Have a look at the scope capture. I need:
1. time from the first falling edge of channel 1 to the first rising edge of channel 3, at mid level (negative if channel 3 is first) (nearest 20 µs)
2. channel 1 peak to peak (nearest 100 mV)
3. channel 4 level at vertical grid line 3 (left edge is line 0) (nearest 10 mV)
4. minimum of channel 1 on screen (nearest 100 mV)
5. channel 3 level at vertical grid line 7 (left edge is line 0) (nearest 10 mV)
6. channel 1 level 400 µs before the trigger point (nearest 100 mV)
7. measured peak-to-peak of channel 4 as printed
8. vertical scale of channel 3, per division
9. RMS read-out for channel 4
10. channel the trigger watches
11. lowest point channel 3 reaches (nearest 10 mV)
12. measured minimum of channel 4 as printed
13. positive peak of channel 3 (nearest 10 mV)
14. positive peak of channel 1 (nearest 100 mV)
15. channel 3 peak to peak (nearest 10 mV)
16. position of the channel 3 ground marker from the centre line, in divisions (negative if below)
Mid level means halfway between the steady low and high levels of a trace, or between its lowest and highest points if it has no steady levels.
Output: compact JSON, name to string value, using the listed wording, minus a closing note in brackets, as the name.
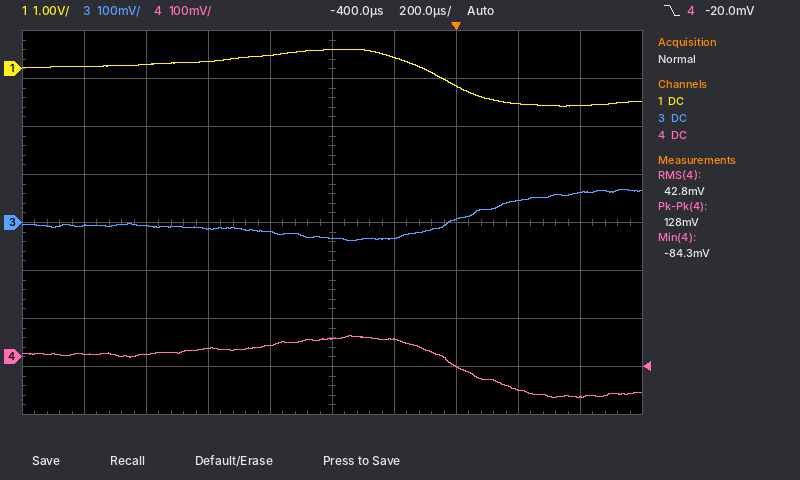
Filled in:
{"time from the first falling edge of channel 1 to the first rising edge of channel 3, at mid level (negative if channel 3 is first)": "+100 µs", "channel 1 peak to peak": "1.2 V", "channel 4 level at vertical grid line 3 (left edge is line 0)": "20 mV", "minimum of channel 1 on screen": "-800 mV", "channel 3 level at vertical grid line 7 (left edge is line 0)": "10 mV", "channel 1 level 400 µs before the trigger point": "400 mV", "measured peak-to-peak of channel 4 as printed": "128 mV", "vertical scale of channel 3, per division": "100 mV", "RMS read-out for channel 4": "42.8 mV", "channel the trigger watches": "channel 4", "lowest point channel 3 reaches": "-40 mV", "measured minimum of channel 4 as printed": "-84.3 mV", "positive peak of channel 3": "70 mV", "positive peak of channel 1": "400 mV", "channel 3 peak to peak": "110 mV", "position of the channel 3 ground marker from the centre line, in divisions": "0.0 div"}
